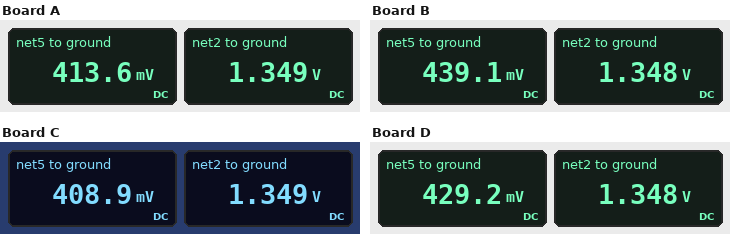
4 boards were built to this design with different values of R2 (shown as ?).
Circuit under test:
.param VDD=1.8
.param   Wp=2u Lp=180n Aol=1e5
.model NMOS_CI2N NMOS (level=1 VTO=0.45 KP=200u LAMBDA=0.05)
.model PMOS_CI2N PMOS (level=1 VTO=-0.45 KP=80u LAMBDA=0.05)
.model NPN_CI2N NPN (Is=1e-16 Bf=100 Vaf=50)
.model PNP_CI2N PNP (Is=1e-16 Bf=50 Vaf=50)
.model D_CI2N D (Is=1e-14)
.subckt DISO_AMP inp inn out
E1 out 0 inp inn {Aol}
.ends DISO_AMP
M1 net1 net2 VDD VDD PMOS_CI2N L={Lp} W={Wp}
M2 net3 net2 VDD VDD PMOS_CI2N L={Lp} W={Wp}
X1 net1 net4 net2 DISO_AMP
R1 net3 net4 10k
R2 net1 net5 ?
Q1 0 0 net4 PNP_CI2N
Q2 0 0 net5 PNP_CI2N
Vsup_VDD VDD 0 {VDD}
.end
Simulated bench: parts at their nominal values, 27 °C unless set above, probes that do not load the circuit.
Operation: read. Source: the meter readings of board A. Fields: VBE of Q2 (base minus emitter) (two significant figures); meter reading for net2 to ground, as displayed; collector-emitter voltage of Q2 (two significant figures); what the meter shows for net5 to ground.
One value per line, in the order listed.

-410 mV
1.349 V
-410 mV
413.6 mV
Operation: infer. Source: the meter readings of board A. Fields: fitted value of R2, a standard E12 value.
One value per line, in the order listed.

15 kΩ
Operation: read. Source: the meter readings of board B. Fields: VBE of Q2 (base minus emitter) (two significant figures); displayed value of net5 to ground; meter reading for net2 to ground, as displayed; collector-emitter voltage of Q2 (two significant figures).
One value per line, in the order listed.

-440 mV
439.1 mV
1.348 V
-440 mV
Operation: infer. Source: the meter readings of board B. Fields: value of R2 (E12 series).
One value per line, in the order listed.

5.6 kΩ
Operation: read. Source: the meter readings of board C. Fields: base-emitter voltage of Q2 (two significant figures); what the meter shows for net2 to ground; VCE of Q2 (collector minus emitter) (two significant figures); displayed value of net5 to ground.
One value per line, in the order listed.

-410 mV
1.349 V
-410 mV
408.9 mV
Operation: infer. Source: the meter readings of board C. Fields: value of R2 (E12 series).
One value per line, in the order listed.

18 kΩ
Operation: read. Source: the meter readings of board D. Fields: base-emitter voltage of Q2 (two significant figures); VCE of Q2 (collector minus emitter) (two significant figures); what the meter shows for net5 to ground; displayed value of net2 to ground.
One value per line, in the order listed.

-430 mV
-430 mV
429.2 mV
1.348 V
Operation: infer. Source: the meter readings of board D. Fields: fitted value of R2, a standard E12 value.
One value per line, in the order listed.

8.2 kΩ
